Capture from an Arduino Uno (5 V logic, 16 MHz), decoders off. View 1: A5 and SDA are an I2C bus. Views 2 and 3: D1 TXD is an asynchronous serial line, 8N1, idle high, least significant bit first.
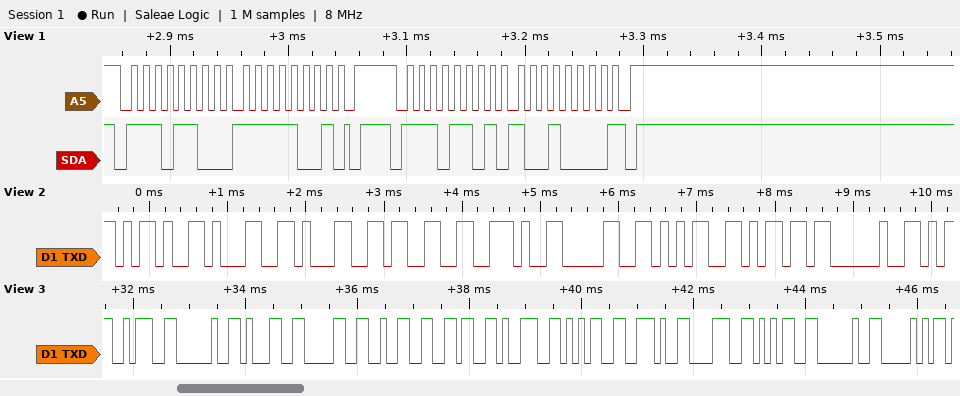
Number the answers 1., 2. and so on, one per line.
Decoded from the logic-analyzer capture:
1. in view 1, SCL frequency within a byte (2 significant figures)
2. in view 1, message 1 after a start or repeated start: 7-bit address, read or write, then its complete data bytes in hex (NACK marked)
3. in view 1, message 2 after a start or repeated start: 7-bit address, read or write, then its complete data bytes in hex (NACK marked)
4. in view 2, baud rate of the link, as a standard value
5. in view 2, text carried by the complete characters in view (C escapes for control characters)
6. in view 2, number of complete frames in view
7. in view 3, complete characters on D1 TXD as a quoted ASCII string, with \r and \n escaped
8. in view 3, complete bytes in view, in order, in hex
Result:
1. 100 kHz
2. 0x76 write: F9
3. 0x76 read: 90 NACK
4. 9600 baud
5. "-113.05m "
6. 9
7. ": 102695.85 P"
8. 3A 20 31 30 32 36 39 35 2E 38 35 20 50
